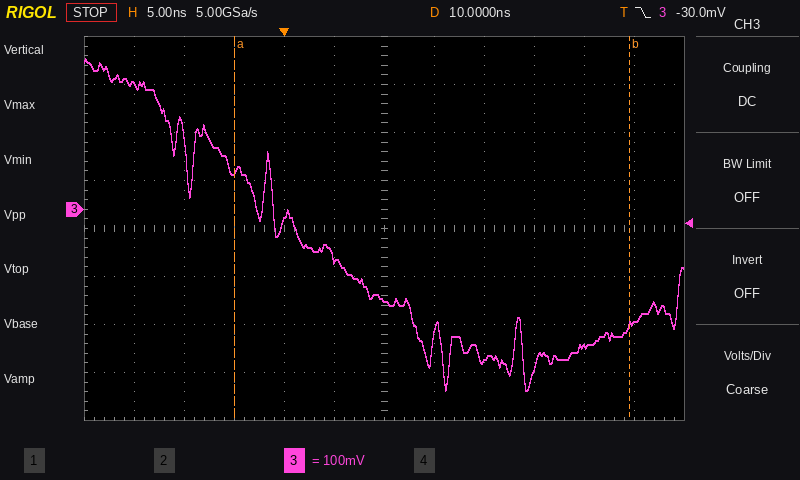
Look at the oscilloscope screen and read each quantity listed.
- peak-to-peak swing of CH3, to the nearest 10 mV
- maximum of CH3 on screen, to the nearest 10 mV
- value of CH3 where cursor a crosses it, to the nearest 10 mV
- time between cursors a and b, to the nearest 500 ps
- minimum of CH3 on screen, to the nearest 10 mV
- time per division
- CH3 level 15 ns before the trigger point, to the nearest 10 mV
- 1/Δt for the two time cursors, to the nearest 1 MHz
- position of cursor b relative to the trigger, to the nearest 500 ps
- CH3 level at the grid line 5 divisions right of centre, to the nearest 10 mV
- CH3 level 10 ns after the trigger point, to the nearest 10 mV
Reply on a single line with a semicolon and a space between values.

690 mV; 310 mV; 80 mV; 39.5 ns; -380 mV; 5 ns; 260 mV; 25 MHz; +34.5 ns; -240 mV; -190 mV
